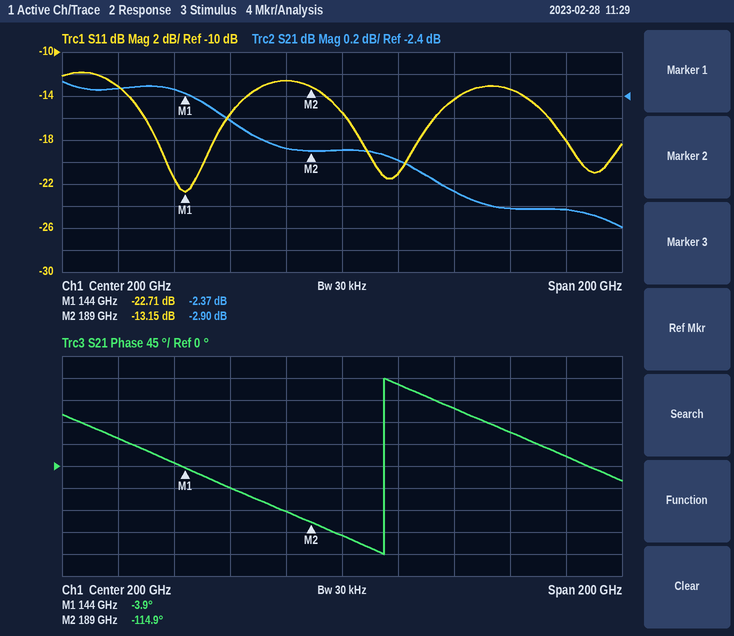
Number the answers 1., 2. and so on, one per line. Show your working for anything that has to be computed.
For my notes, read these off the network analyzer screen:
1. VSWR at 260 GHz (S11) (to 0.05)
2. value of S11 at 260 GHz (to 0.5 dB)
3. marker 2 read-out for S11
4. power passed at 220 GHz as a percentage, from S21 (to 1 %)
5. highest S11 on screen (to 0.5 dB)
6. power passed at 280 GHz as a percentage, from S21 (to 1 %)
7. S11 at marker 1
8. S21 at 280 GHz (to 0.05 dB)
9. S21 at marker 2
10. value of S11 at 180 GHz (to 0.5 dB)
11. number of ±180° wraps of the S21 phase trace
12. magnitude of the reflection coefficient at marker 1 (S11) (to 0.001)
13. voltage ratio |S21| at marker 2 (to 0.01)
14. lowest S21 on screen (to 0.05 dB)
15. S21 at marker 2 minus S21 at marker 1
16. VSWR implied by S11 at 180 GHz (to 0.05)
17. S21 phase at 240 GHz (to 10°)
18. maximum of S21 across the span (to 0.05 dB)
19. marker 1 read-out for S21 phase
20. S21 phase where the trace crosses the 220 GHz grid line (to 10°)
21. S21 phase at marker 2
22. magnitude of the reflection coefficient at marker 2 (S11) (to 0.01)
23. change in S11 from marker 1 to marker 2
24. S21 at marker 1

1. |Γ| = 10^(-13.5/20) = 0.2113; VSWR = (1 + 0.2113)/(1 − 0.2113) ≈ 1.54, so 1.55 to the nearest 0.05
2. -13.5 dB
3. -13.15 dB
4. 10^(-3/10) ≈ 50 %
5. -12.0 dB
6. 10^(-3.45/10) ≈ 45 %
7. -22.71 dB
8. -3.45 dB
9. -2.90 dB
10. -12.5 dB
11. 1
12. 10^(-22.71/20) ≈ 0.073
13. 10^(-2.9/20) ≈ 0.72
14. -3.60 dB
15. -2.9 − (-2.37) = -0.53 dB
16. |Γ| = 10^(-12.5/20) = 0.2371; VSWR = (1 + 0.2371)/(1 − 0.2371) ≈ 1.62, so 1.60 to the nearest 0.05
17. 120°
18. -2.25 dB
19. -3.9°
20. 170°
21. -114.9°
22. 10^(-13.15/20) ≈ 0.22
23. -13.15 − (-22.71) = 9.56 dB
24. -2.37 dB
